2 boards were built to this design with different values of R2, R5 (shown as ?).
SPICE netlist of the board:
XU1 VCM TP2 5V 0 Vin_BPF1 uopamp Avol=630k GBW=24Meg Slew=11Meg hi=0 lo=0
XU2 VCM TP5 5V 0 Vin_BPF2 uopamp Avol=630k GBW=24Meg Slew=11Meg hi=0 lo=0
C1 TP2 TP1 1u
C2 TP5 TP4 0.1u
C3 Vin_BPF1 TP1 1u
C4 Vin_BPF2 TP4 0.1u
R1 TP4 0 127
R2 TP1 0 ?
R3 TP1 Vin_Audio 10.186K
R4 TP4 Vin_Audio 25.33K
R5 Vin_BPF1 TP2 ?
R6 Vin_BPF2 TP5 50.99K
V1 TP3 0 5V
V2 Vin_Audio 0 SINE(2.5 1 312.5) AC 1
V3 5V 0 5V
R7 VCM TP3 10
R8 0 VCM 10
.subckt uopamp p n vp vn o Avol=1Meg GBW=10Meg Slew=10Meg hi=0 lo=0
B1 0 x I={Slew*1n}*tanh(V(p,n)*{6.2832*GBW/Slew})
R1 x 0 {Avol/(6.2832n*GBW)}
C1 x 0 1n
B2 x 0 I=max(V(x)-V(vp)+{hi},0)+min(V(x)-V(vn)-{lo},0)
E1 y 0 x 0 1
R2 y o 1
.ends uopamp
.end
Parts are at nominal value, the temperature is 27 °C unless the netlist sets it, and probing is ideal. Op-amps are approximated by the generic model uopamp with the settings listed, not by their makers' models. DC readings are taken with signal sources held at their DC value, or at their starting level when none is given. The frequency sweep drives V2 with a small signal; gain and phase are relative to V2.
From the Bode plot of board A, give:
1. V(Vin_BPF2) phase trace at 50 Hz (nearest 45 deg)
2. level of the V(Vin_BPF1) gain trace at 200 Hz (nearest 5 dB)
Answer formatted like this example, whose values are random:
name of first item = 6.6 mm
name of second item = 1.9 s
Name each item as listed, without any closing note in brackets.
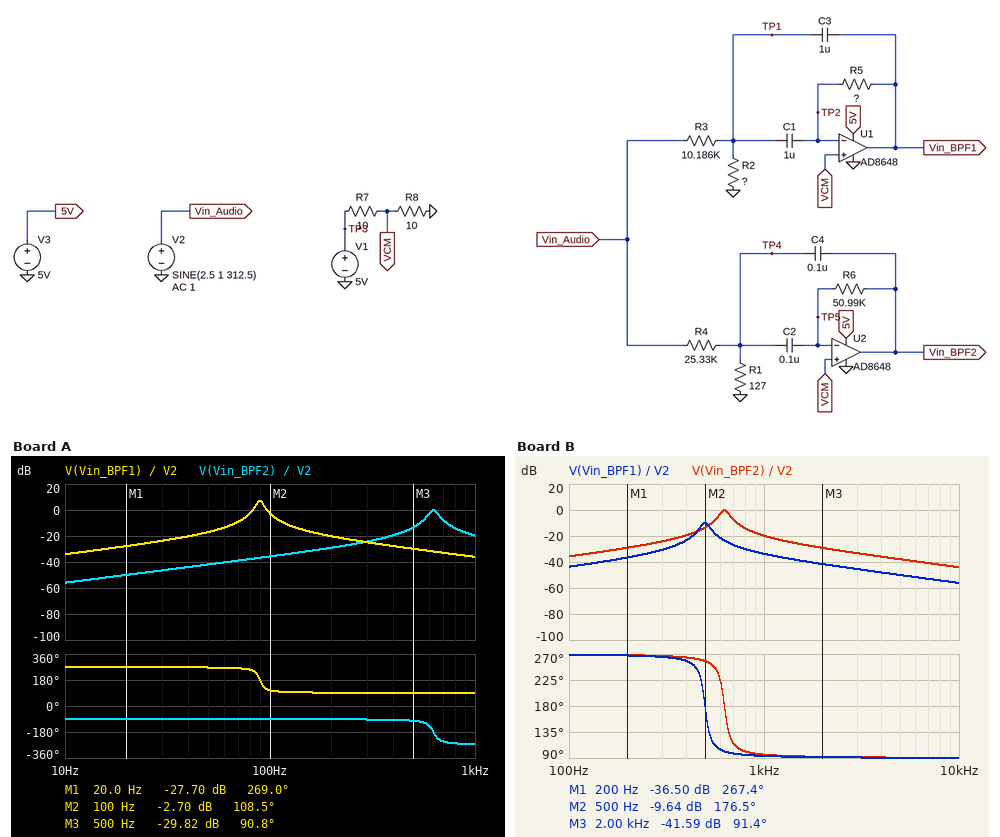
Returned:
V(Vin_BPF2) phase trace at 50 Hz = -90 deg
level of the V(Vin_BPF1) gain trace at 200 Hz = -20 dB
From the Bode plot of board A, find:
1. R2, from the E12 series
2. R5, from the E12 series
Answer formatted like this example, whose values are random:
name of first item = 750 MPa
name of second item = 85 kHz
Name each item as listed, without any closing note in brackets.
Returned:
R2, from the E12 series = 68 Ω
R5, from the E12 series = 47 kΩ
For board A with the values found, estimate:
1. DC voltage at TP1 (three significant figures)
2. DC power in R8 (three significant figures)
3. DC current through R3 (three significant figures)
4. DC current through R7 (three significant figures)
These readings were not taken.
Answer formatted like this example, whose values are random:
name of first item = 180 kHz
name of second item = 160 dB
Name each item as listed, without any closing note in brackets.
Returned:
DC voltage at TP1 = 16.6 mV
DC power in R8 = 625 mW
DC current through R3 = 244 µA
DC current through R7 = 250 mA
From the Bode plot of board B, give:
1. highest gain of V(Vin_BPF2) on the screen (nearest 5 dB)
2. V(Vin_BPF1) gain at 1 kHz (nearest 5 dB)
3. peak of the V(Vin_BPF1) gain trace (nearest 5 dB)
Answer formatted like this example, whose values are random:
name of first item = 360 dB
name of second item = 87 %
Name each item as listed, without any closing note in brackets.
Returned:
highest gain of V(Vin_BPF2) on the screen = 0 dB
V(Vin_BPF1) gain at 1 kHz = -35 dB
peak of the V(Vin_BPF1) gain trace = -10 dB
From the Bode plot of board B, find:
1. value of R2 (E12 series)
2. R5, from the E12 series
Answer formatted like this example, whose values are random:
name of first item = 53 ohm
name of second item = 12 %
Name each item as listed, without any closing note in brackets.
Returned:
value of R2 = 15 Ω
R5, from the E12 series = 6.8 kΩ
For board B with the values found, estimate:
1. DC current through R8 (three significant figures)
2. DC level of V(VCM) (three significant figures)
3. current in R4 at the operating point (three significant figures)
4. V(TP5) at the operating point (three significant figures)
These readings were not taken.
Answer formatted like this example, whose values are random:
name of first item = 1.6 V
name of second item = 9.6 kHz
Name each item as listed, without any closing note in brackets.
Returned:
DC current through R8 = 250 mA
DC level of V(VCM) = 2.50 V
current in R4 at the operating point = 98.2 µA
V(TP5) at the operating point = 2.50 V
